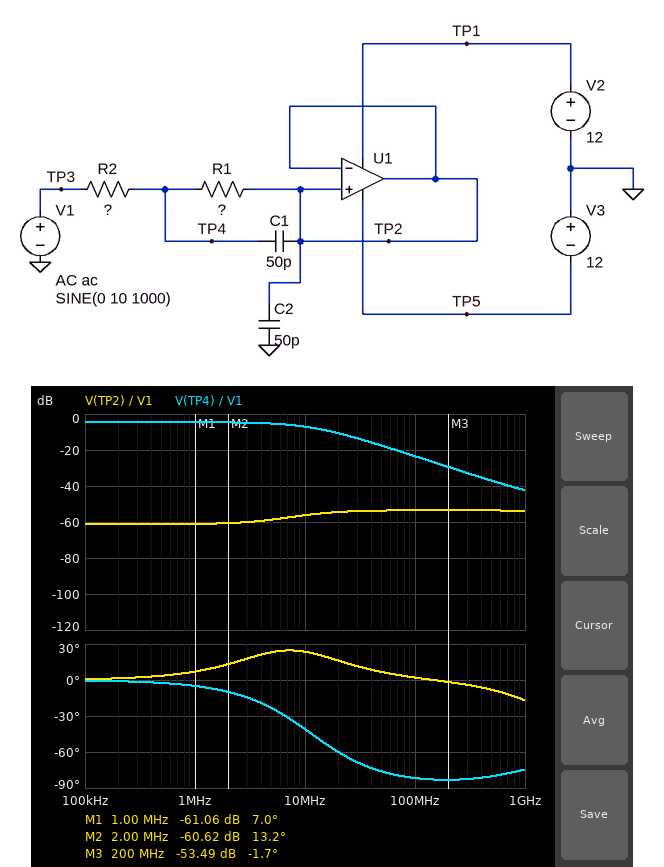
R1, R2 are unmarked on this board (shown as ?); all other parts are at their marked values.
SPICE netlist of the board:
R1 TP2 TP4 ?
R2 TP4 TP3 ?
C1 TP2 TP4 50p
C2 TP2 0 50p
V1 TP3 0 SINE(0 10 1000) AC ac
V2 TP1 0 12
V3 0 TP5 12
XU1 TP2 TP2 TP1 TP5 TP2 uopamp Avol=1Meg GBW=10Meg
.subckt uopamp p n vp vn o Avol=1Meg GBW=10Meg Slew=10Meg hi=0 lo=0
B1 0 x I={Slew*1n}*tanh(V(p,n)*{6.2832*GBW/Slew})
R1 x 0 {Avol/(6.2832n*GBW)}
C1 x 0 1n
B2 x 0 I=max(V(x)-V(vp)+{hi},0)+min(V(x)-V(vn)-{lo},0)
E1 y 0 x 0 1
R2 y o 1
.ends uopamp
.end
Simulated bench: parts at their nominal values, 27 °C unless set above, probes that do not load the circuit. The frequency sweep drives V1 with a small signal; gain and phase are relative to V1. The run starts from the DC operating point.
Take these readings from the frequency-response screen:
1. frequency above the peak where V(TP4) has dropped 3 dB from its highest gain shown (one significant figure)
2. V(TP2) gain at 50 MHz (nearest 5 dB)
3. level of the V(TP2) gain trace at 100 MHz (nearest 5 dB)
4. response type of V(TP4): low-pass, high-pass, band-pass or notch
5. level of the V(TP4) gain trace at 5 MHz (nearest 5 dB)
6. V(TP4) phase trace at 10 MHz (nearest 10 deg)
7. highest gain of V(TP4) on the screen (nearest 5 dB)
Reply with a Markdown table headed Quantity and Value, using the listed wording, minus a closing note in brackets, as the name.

| Quantity | Value |
|---|---|
| frequency above the peak where V(TP4) has dropped 3 dB from its highest gain shown | 10 MHz |
| V(TP2) gain at 50 MHz | -55 dB |
| level of the V(TP2) gain trace at 100 MHz | -55 dB |
| response type of V(TP4): low-pass, high-pass, band-pass or notch | low-pass |
| level of the V(TP4) gain trace at 5 MHz | -5 dB |
| V(TP4) phase trace at 10 MHz | -40 deg |
| highest gain of V(TP4) on the screen | -5 dB |
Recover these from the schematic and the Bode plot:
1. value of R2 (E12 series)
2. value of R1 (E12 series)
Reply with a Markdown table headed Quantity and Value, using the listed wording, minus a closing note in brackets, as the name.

| Quantity | Value |
|---|---|
| value of R2 | 470 Ω |
| value of R1 | 680 Ω |
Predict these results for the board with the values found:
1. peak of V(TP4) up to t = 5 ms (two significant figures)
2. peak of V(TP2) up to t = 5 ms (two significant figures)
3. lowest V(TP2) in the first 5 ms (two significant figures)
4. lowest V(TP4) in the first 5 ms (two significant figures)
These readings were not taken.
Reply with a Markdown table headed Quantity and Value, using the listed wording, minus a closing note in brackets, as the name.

| Quantity | Value |
|---|---|
| peak of V(TP4) up to t = 5 ms | 5.9 V |
| peak of V(TP2) up to t = 5 ms | 8.7 mV |
| lowest V(TP2) in the first 5 ms | -8.7 mV |
| lowest V(TP4) in the first 5 ms | -5.9 V |
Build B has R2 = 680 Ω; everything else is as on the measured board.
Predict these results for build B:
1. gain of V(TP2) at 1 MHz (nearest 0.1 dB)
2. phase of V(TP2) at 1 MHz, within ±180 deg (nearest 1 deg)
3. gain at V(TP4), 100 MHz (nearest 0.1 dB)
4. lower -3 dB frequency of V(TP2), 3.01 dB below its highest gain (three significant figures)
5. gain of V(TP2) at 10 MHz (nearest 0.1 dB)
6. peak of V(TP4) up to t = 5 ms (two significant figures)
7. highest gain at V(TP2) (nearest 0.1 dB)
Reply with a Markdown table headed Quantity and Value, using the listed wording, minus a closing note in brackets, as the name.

| Quantity | Value |
|---|---|
| gain of V(TP2) at 1 MHz | -62.5 dB |
| phase of V(TP2) at 1 MHz, within ±180 deg | 6 deg |
| gain at V(TP4), 100 MHz | -26.6 dB |
| lower -3 dB frequency of V(TP2), 3.01 dB below its highest gain | 6.56 MHz |
| gain of V(TP2) at 10 MHz | -58.5 dB |
| peak of V(TP4) up to t = 5 ms | 5.0 V |
| highest gain at V(TP2) | -56.7 dB |
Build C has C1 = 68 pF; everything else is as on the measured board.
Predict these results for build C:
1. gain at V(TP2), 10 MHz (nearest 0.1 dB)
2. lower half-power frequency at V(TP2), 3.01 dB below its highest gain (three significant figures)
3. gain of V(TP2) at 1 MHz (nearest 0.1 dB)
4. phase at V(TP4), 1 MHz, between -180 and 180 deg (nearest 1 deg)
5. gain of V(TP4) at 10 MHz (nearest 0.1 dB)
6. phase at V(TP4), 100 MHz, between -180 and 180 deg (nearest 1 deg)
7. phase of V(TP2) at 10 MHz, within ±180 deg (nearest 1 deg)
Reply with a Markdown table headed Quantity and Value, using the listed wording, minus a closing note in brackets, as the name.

| Quantity | Value |
|---|---|
| gain at V(TP2), 10 MHz | -55.3 dB |
| lower half-power frequency at V(TP2), 3.01 dB below its highest gain | 6.82 MHz |
| gain of V(TP2) at 1 MHz | -60.9 dB |
| phase at V(TP4), 1 MHz, between -180 and 180 deg | -7 deg |
| gain of V(TP4) at 10 MHz | -8.4 dB |
| phase at V(TP4), 100 MHz, between -180 and 180 deg | -83 deg |
| phase of V(TP2) at 10 MHz, within ±180 deg | 21 deg |
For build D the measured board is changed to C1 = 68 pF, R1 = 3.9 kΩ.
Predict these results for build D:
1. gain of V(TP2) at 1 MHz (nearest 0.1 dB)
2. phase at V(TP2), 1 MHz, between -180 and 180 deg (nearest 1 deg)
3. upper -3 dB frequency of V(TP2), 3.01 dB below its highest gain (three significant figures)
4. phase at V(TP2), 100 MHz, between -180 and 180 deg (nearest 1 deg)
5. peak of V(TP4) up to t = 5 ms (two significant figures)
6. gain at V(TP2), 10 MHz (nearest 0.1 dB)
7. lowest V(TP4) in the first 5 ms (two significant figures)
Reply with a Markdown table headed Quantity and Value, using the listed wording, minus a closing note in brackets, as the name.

| Quantity | Value |
|---|---|
| gain of V(TP2) at 1 MHz | -67.2 dB |
| phase at V(TP2), 1 MHz, between -180 and 180 deg | 49 deg |
| upper -3 dB frequency of V(TP2), 3.01 dB below its highest gain | 3.20 GHz |
| phase at V(TP2), 100 MHz, between -180 and 180 deg | 1 deg |
| peak of V(TP4) up to t = 5 ms | 8.9 V |
| gain at V(TP2), 10 MHz | -54.6 dB |
| lowest V(TP4) in the first 5 ms | -8.9 V |
